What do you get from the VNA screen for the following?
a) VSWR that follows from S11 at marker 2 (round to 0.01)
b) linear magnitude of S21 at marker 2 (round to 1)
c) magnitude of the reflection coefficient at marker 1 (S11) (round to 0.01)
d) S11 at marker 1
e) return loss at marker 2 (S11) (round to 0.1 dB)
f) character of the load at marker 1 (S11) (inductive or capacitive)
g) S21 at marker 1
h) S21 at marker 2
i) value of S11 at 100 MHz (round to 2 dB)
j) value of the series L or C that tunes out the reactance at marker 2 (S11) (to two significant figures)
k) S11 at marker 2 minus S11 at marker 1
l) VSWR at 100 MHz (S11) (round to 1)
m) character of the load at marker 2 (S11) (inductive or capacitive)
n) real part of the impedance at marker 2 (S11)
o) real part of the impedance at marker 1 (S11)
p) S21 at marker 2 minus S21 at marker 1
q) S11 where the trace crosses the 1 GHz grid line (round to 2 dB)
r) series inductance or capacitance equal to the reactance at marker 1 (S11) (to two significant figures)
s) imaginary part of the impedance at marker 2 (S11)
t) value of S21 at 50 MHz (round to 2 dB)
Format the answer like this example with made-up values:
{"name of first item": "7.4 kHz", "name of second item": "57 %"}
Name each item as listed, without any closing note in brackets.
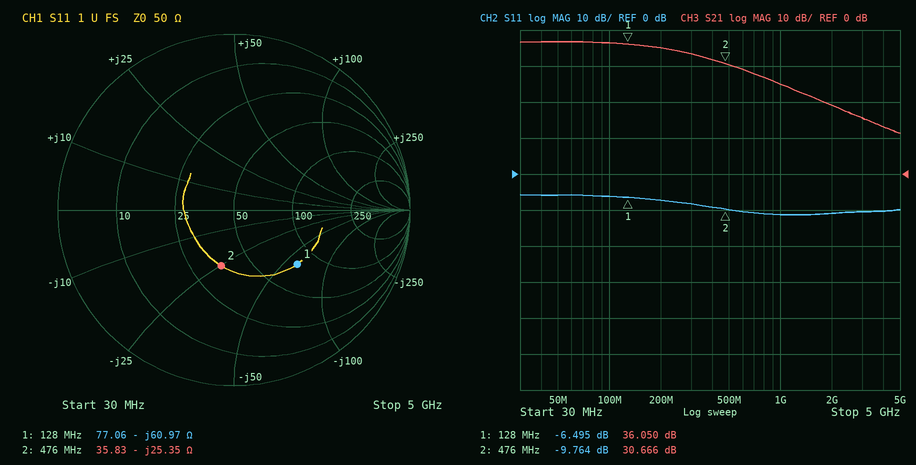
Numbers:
{"VSWR that follows from S11 at marker 2": "1.96", "linear magnitude of S21 at marker 2": "34", "magnitude of the reflection coefficient at marker 1 (S11)": "0.47", "S11 at marker 1": "-6.495 dB", "return loss at marker 2 (S11)": "9.8 dB", "character of the load at marker 1 (S11)": "capacitive", "S21 at marker 1": "36.050 dB", "S21 at marker 2": "30.666 dB", "value of S11 at 100 MHz": "-6 dB", "value of the series L or C that tunes out the reactance at marker 2 (S11)": "8.5 nH", "S11 at marker 2 minus S11 at marker 1": "-3.269 dB", "VSWR at 100 MHz (S11)": "3", "character of the load at marker 2 (S11)": "capacitive", "real part of the impedance at marker 2": "35.83 Ω", "real part of the impedance at marker 1": "77.06 Ω", "S21 at marker 2 minus S21 at marker 1": "-5.384 dB", "S11 where the trace crosses the 1 GHz grid line": "-12 dB", "series inductance or capacitance equal to the reactance at marker 1 (S11)": "20 pF", "imaginary part of the impedance at marker 2": "-25.35 Ω", "value of S21 at 50 MHz": "36 dB"}
